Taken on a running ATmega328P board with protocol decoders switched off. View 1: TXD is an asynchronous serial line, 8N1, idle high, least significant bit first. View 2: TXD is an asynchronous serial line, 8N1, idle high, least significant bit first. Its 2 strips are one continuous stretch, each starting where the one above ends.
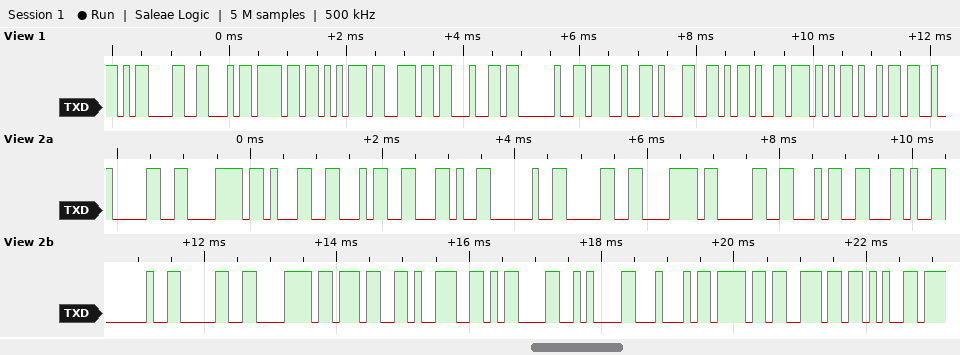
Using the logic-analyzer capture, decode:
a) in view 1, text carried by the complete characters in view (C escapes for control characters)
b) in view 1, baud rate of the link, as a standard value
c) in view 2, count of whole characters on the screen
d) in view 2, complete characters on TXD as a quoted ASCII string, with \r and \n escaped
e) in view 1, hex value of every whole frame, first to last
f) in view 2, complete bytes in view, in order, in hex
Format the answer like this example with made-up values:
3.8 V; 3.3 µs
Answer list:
"\rFound '1-Wi"; 9600 baud; 22; "0x14, 0x04, 0x79\r\nDone"; 0x0D 0x46 0x6F 0x75 0x6E 0x64 0x20 0x27 0x31 0x2D 0x57 0x69; 30 78 31 34 2C 20 30 78 30 34 2C 20 30 78 37 39 0D 0A 44 6F 6E 65
